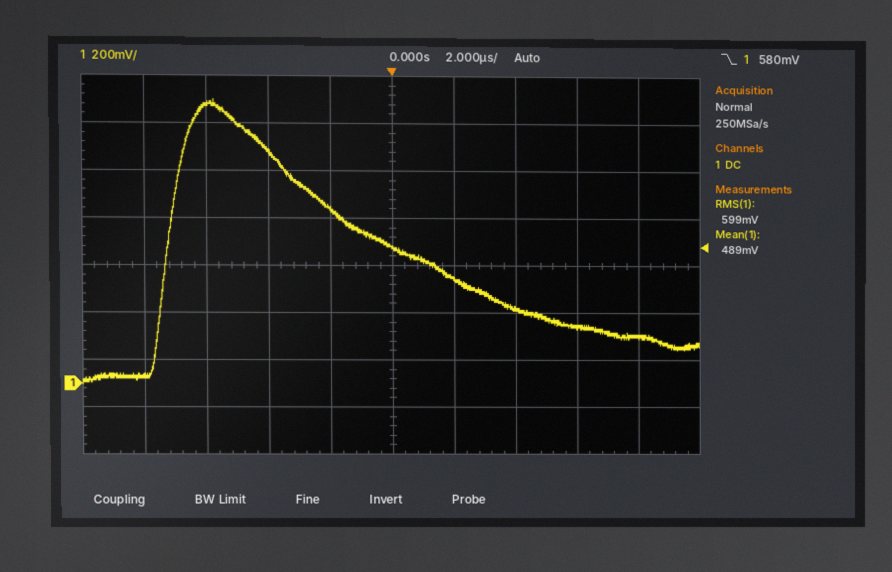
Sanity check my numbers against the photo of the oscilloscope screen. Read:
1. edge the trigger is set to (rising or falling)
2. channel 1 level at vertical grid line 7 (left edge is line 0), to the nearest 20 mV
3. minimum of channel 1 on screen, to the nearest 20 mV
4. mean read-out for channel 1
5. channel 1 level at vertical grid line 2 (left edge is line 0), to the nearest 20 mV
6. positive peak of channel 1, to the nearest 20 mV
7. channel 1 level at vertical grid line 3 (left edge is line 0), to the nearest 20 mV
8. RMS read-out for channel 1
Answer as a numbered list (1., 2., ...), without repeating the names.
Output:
1. falling
2. 320 mV
3. 0 mV
4. 489 mV
5. 1.18 V
6. 1.20 V
7. 980 mV
8. 599 mV
